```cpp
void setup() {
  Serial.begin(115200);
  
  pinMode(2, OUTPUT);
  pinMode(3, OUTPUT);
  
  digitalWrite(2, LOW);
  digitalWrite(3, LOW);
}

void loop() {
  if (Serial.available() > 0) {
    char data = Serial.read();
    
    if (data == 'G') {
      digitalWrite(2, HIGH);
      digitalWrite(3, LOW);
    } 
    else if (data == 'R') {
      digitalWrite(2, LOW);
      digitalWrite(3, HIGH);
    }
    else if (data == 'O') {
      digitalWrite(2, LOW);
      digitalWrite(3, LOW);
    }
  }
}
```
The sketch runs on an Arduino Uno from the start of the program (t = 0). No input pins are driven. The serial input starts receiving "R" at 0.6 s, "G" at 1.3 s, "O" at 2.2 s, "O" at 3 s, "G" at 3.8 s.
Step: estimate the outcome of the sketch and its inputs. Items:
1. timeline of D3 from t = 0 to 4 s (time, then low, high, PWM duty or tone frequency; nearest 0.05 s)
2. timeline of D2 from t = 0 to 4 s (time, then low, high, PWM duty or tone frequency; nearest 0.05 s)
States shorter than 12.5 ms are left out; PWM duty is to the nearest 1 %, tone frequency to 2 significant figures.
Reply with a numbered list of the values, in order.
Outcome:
1. 0 s low; 0.6 s high; 1.3 s low
2. 0 s low; 1.3 s high; 2.2 s low; 3.8 s high
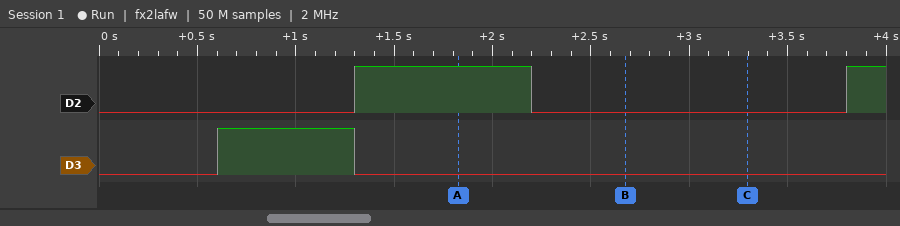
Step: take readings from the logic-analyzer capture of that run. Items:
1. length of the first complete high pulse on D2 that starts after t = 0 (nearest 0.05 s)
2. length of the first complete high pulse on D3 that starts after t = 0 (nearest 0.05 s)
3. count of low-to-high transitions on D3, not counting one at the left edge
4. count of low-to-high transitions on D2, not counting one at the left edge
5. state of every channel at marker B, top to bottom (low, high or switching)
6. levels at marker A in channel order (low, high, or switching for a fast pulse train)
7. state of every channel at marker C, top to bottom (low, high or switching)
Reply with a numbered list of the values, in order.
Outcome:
1. 0.90 s
2. 0.70 s
3. 1
4. 2
5. D2 low, D3 low
6. D2 high, D3 low
7. D2 low, D3 low
